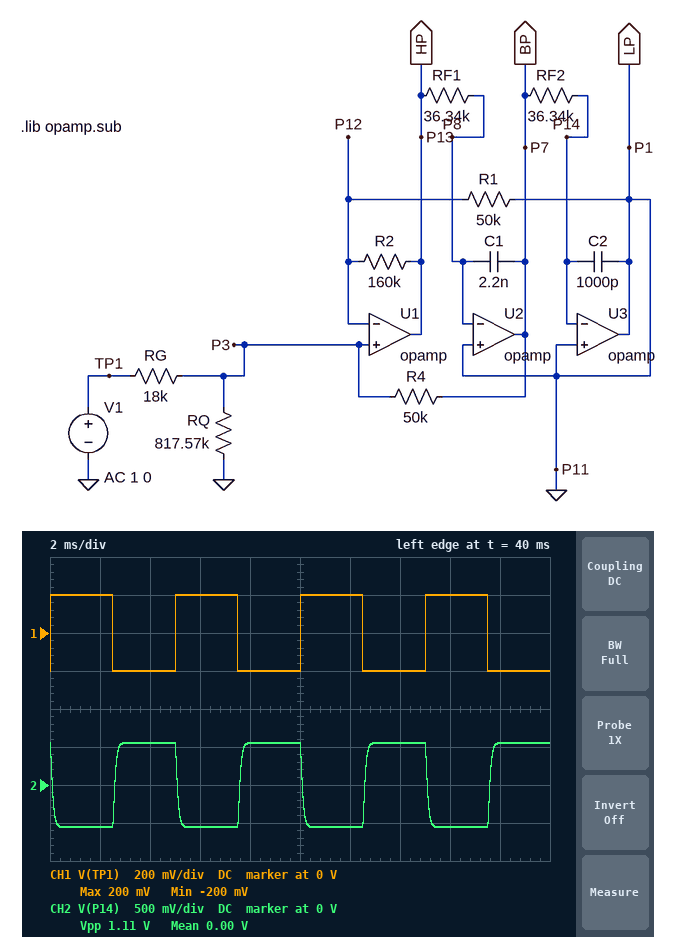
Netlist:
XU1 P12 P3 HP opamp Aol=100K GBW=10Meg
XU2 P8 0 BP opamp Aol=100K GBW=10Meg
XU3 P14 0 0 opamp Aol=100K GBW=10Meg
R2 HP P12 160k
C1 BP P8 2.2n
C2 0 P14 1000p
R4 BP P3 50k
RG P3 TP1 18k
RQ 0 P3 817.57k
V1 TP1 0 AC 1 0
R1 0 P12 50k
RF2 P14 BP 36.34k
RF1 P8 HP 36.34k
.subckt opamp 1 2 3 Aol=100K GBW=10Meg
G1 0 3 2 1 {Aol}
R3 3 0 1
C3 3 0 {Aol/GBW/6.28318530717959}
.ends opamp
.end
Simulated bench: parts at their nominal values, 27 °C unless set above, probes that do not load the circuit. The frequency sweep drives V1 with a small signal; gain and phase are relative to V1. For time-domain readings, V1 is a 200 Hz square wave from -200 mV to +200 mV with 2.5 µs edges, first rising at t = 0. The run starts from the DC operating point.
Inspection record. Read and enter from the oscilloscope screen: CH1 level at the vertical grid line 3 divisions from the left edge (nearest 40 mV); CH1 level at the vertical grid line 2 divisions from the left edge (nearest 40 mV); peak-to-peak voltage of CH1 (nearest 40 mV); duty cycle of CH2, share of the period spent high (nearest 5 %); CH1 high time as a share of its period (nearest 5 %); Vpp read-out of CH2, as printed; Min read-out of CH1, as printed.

200 mV
-200 mV
400 mV
50 %
50 %
1.11 V
-200 mV
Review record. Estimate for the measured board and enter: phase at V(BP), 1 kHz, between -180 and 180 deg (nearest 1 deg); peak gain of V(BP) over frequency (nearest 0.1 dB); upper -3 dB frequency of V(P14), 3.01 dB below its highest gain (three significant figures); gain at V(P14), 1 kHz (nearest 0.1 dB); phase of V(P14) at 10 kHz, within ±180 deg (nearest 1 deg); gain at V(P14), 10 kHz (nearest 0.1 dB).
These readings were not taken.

155 deg
8.9 dB
1.83 kHz
7.8 dB
36 deg
-12.5 dB
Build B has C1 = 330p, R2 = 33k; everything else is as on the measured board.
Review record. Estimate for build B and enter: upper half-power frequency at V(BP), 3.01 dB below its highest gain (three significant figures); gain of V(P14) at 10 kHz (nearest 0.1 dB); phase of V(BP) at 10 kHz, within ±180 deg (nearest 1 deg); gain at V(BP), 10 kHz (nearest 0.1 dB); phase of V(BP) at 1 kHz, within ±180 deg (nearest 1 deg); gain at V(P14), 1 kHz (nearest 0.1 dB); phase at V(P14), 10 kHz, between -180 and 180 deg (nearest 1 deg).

5.74 kHz
-5.1 dB
120 deg
2.8 dB
170 deg
8.5 dB
53 deg
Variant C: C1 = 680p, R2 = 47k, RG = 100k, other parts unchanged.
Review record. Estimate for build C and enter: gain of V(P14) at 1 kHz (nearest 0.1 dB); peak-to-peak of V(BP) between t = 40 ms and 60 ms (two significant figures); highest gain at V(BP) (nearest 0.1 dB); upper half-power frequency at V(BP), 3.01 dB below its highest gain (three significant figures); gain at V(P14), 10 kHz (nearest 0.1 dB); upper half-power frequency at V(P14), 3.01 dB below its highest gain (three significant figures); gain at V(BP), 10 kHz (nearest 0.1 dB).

-6.3 dB
200 mV
-6.0 dB
8.02 kHz
-18.0 dB
3.58 kHz
-10.1 dB
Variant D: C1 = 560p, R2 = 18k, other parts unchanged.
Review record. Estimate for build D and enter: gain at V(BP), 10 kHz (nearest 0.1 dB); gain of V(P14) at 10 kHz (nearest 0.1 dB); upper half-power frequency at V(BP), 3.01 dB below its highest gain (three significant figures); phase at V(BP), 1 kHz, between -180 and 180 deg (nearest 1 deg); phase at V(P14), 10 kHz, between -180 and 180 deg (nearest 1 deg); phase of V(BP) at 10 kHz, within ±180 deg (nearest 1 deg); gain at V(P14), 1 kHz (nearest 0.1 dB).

-2.6 dB
-10.5 dB
2.77 kHz
160 deg
39 deg
105 deg
8.1 dB
